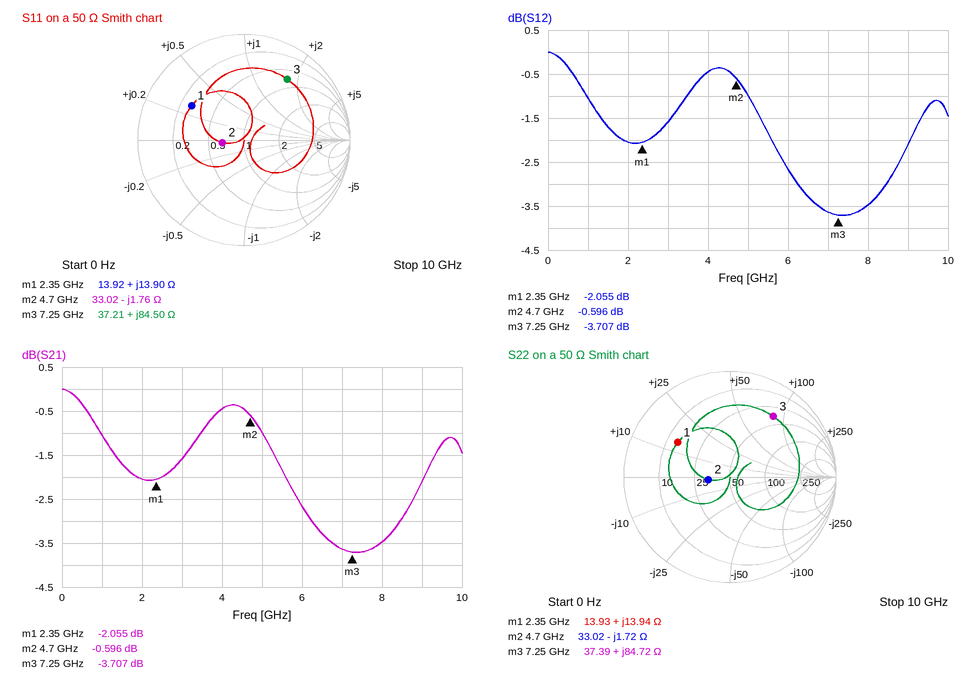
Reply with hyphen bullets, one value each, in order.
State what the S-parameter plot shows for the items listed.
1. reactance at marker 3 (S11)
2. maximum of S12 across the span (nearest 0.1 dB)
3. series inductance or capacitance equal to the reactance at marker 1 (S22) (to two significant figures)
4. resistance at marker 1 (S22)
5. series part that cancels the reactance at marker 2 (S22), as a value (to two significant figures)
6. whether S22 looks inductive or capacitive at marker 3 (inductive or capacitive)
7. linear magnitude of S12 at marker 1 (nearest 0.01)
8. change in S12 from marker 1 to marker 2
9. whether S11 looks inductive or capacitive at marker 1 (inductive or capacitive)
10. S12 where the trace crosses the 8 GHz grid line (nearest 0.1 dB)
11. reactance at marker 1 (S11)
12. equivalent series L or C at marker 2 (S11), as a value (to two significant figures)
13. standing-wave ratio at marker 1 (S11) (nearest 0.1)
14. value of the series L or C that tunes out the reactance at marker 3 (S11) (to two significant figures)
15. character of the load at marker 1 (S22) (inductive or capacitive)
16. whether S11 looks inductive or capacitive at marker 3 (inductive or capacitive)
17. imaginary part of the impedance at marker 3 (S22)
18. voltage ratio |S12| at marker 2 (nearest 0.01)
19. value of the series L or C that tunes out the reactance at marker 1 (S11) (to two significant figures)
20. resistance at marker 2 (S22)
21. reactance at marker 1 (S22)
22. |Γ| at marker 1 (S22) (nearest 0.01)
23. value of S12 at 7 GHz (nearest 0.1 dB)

- +84.50 Ω
- 0.0 dB
- 940 pH
- 13.93 Ω
- 58 pH
- inductive
- 0.79
- 1.459 dB
- inductive
- -3.5 dB
- +13.90 Ω
- 19 pF
- 3.9
- 260 fF
- inductive
- inductive
- +84.72 Ω
- 0.93
- 4.9 pF
- 33.02 Ω
- +13.94 Ω
- 0.59
- -3.6 dB
